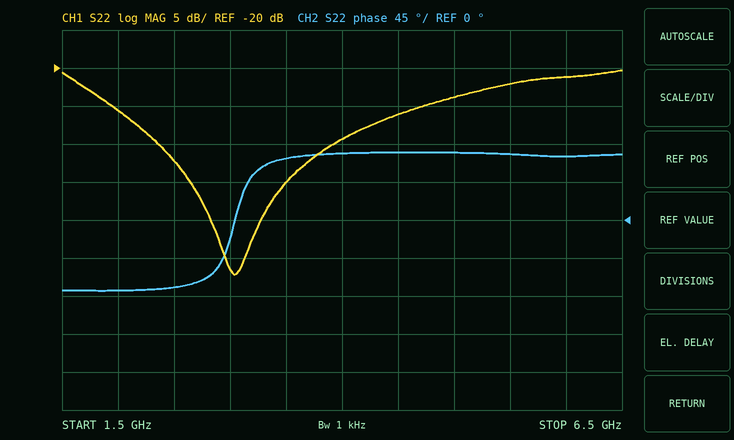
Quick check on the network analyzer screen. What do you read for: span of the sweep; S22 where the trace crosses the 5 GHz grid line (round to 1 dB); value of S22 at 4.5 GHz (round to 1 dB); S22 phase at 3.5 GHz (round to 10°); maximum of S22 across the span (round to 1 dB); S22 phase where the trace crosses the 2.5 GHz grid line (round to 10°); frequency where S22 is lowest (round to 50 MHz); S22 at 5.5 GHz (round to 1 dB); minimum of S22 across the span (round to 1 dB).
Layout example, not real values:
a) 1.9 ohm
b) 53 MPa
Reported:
a) 5 GHz
b) -24 dB
c) -26 dB
d) 70°
e) -20 dB
f) -80°
g) 3.05 GHz
h) -22 dB
i) -47 dB
